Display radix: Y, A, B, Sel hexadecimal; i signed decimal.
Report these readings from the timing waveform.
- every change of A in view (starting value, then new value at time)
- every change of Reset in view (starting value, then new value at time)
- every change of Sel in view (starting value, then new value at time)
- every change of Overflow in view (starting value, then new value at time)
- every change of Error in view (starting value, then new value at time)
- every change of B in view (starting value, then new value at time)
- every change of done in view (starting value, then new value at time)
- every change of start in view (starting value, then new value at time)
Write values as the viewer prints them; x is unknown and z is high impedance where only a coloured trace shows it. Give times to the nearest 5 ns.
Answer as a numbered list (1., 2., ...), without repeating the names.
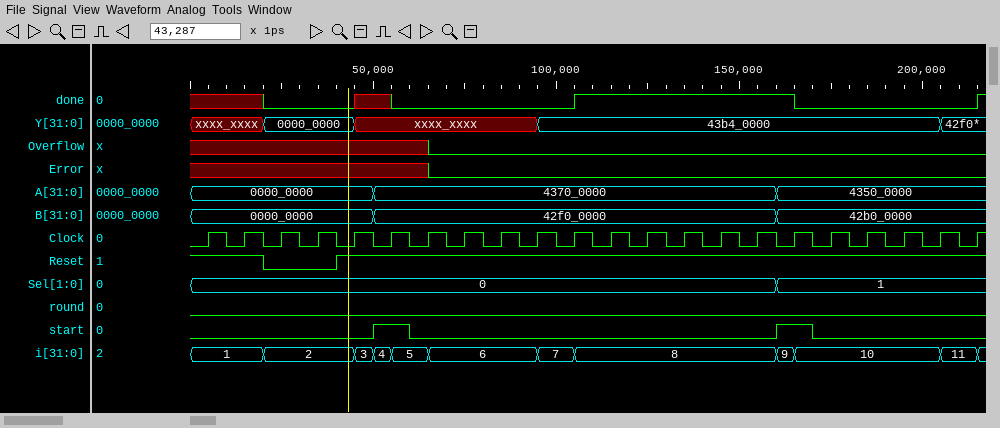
1. 0000_0000, 4370_0000 at 50 ns, 4350_0000 at 160 ns
2. 1, 0 at 20 ns, 1 at 40 ns
3. 0, 1 at 160 ns
4. x, 0 at 65 ns
5. x, 0 at 65 ns
6. 0000_0000, 42f0_0000 at 50 ns, 42b0_0000 at 160 ns
7. x, 0 at 20 ns, x at 45 ns, 0 at 55 ns, 1 at 105 ns, 0 at 165 ns, 1 at 215 ns
8. 0, 1 at 50 ns, 0 at 60 ns, 1 at 160 ns, 0 at 170 ns
